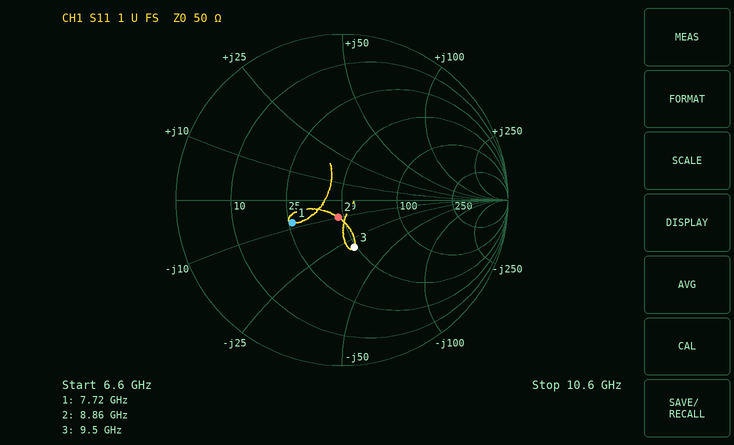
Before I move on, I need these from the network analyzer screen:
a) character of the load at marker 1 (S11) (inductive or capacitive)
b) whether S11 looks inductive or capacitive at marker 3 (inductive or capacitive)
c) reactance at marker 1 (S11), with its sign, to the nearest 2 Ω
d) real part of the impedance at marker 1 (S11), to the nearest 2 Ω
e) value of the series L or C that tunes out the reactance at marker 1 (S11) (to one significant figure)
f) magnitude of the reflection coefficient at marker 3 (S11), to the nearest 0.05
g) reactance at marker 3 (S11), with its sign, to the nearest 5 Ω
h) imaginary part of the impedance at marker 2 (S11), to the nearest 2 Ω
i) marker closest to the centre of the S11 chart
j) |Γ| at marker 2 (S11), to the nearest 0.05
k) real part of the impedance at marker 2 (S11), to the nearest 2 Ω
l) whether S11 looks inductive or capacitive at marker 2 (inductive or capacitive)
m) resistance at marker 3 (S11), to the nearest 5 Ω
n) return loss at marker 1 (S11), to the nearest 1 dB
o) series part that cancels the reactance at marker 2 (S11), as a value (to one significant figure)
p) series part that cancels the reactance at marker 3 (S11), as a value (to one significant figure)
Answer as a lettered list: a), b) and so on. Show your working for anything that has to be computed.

a) capacitive
b) capacitive
c) -8 Ω
d) 26 Ω
e) L = 8 Ω/(2π × 7.72 GHz) ≈ 165 pH, so 200 pH to one significant figure
f) 0.30
g) -30 Ω
h) -10 Ω
i) marker 2
j) 0.10
k) 46 Ω
l) capacitive
m) 50 Ω
n) 10 dB
o) L = 10 Ω/(2π × 8.86 GHz) ≈ 180 pH, so 200 pH to one significant figure
p) L = 30 Ω/(2π × 9.5 GHz) ≈ 503 pH, so 500 pH to one significant figure
